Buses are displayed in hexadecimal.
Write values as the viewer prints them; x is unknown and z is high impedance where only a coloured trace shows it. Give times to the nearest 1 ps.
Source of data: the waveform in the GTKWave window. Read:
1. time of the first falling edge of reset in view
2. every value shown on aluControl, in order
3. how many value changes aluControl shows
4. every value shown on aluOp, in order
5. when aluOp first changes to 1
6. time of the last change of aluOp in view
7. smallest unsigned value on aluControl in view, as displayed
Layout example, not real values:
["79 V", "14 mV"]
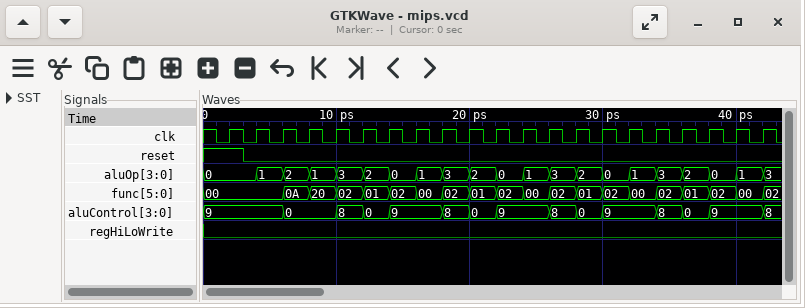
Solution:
["3 ps", "9, 0, 8, 0, 9, 8, 0, 9, 8, 0, 9, 8, 0, 9, 8", "14", "0, 1, 2, 1, 3, 2, 0, 1, 3, 2, 0, 1, 3, 2, 0, 1, 3, 2, 0, 1, 3", "4 ps", "42 ps", "0"]
